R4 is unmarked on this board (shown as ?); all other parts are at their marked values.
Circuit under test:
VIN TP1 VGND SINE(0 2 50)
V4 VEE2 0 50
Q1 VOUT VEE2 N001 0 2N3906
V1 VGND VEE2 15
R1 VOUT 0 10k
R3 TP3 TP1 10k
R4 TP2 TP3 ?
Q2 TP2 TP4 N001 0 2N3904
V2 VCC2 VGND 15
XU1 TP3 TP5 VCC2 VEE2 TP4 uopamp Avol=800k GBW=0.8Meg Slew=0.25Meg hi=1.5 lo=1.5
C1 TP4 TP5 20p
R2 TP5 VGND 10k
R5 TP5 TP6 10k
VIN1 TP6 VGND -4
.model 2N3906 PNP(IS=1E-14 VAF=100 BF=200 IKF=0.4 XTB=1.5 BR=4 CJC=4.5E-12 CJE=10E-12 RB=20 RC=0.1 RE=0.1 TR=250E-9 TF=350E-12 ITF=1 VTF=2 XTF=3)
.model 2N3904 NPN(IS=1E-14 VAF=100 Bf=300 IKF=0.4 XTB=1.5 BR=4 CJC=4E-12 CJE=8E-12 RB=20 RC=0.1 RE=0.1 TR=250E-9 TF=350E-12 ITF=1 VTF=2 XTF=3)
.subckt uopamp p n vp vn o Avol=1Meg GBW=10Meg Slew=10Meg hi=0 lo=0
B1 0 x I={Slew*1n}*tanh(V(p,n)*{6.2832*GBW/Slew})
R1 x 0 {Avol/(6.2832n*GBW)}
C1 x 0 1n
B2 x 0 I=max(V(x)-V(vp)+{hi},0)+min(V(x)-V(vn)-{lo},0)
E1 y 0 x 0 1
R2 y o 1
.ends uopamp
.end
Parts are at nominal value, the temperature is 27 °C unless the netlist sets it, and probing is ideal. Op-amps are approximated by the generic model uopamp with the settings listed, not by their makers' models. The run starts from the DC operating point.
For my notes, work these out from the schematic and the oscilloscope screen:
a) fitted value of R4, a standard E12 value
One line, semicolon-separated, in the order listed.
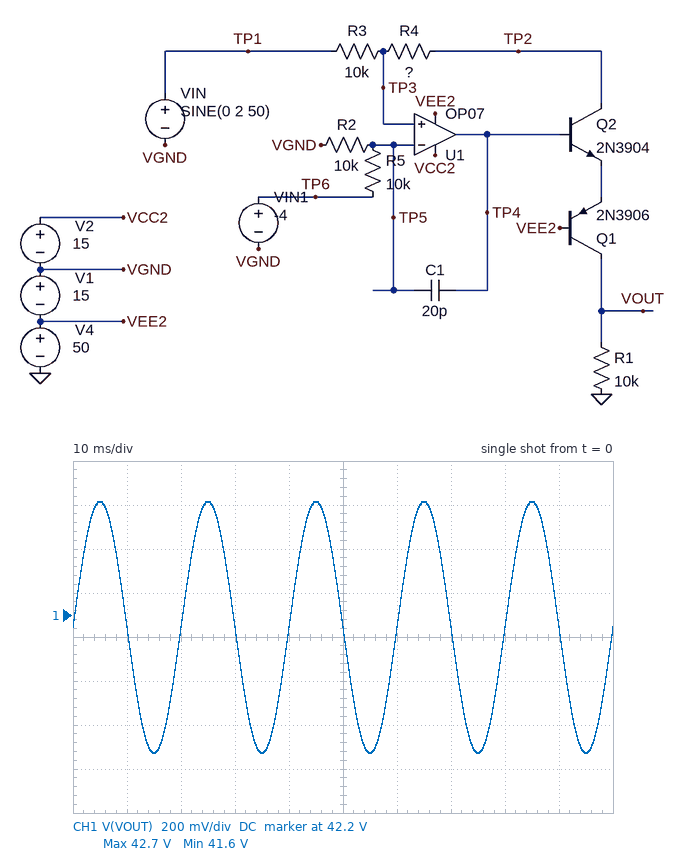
15 kΩ
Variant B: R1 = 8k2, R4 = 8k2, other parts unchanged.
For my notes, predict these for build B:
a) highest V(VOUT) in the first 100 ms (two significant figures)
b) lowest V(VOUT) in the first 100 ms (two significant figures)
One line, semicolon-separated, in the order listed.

37 V; 36 V
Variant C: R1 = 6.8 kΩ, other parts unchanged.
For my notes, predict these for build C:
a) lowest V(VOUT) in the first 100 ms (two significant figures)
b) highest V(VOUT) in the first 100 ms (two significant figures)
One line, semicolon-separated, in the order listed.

29 V; 30 V
